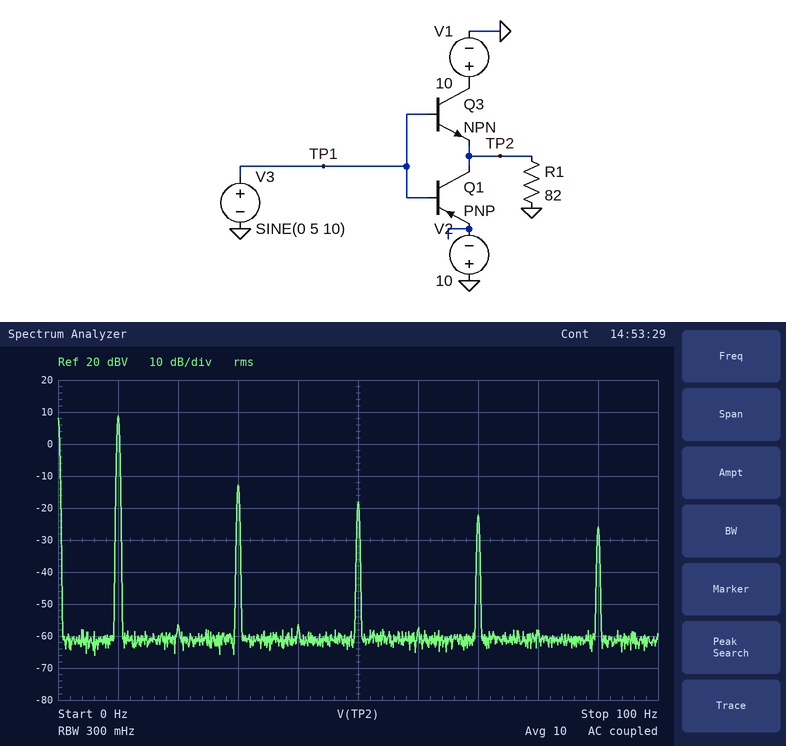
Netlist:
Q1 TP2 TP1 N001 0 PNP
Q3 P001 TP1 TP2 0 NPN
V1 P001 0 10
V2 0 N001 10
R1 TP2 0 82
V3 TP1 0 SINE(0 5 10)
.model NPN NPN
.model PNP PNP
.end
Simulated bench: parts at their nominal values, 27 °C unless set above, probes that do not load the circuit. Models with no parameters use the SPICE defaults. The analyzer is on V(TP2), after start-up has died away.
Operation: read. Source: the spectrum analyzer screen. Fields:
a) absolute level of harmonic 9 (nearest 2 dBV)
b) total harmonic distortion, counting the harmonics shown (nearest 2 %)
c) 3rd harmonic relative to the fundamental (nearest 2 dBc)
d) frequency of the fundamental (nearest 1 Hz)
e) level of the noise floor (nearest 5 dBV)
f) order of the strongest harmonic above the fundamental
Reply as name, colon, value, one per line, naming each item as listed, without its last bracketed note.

absolute level of harmonic 9: -26 dBV
total harmonic distortion, counting the harmonics shown: 10 %
3rd harmonic relative to the fundamental: -22 dBc
frequency of the fundamental: 10 Hz
level of the noise floor: -60 dBV
order of the strongest harmonic above the fundamental: 3
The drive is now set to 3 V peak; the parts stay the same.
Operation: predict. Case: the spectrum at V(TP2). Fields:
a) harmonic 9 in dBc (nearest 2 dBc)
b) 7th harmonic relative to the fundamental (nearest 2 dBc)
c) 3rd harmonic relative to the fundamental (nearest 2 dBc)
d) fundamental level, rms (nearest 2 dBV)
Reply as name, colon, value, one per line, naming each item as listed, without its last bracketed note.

harmonic 9 in dBc: -36 dBc
7th harmonic relative to the fundamental: -30 dBc
3rd harmonic relative to the fundamental: -16 dBc
fundamental level, rms: 2 dBV
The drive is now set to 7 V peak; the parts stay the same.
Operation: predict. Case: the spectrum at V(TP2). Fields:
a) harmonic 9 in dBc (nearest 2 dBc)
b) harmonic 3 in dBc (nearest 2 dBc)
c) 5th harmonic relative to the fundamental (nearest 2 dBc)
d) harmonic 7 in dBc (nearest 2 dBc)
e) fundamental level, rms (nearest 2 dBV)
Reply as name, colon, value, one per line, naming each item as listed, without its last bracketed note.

harmonic 9 in dBc: -36 dBc
harmonic 3 in dBc: -24 dBc
5th harmonic relative to the fundamental: -30 dBc
harmonic 7 in dBc: -34 dBc
fundamental level, rms: 12 dBV
